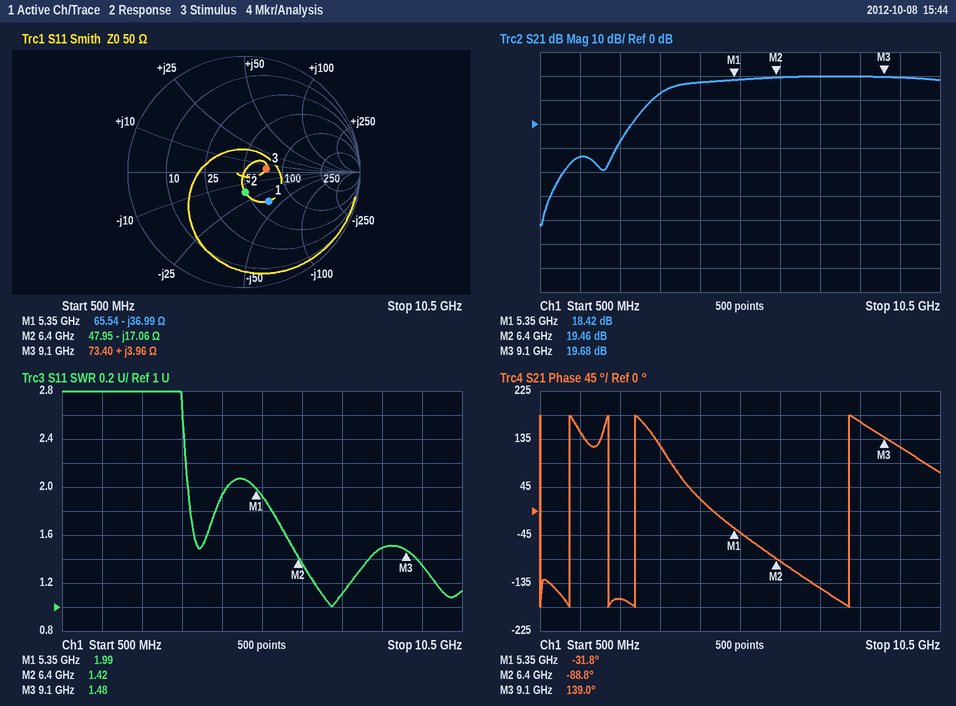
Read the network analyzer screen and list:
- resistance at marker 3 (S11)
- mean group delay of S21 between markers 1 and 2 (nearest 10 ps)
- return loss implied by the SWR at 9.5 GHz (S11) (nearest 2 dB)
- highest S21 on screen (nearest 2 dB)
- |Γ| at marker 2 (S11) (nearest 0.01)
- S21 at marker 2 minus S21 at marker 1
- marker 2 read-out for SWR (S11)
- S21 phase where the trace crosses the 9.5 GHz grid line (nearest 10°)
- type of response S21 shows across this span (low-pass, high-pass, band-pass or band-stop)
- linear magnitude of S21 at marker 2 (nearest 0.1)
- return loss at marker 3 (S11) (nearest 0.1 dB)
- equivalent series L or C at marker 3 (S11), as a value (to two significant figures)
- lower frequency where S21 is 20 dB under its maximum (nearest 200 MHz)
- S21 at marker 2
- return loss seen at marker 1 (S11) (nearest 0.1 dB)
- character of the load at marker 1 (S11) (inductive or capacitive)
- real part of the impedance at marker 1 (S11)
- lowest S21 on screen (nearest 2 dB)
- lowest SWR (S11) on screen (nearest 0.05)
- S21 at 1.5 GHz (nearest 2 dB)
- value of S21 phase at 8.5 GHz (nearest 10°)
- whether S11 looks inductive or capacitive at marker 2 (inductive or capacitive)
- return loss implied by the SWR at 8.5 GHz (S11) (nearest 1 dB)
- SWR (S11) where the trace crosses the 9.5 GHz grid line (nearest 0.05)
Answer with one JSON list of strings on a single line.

["73.40 Ω", "150 ps", "16 dB", "20 dB", "0.17", "1.04 dB", "1.42", "120°", "high-pass", "9.4", "14.3 dB", "69 pH", "2.8 GHz", "19.46 dB", "9.6 dB", "capacitive", "65.54 Ω", "-42 dB", "1.00", "-14 dB", "170°", "capacitive", "14 dB", "1.35"]
